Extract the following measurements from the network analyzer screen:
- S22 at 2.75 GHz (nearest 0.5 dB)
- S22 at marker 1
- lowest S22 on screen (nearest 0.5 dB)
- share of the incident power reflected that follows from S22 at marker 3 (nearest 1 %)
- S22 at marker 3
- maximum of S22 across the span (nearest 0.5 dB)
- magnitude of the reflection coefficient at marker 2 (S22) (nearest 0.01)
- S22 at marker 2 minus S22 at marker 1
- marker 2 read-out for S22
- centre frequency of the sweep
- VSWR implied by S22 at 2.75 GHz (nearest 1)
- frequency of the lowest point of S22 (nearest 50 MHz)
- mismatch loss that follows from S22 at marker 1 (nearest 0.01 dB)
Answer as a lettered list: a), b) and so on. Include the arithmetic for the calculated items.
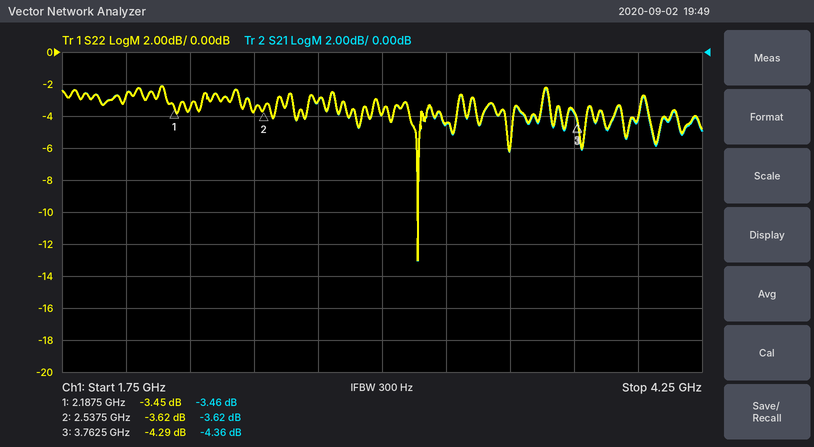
a) -3.0 dB
b) -3.45 dB
c) -13.0 dB
d) 10^(-4.29/10) ≈ 37 %
e) -4.29 dB
f) -2.0 dB
g) 10^(-3.62/20) ≈ 0.66
h) -3.62 − (-3.45) = -0.17 dB
i) -3.62 dB
j) 3 GHz
k) |Γ| = 10^(-3/20) = 0.7079; VSWR = (1 + 0.7079)/(1 − 0.7079) ≈ 6
l) 3.15 GHz
m) −10 log10(1 − 10^(-3.45/10)) ≈ 2.61 dB
